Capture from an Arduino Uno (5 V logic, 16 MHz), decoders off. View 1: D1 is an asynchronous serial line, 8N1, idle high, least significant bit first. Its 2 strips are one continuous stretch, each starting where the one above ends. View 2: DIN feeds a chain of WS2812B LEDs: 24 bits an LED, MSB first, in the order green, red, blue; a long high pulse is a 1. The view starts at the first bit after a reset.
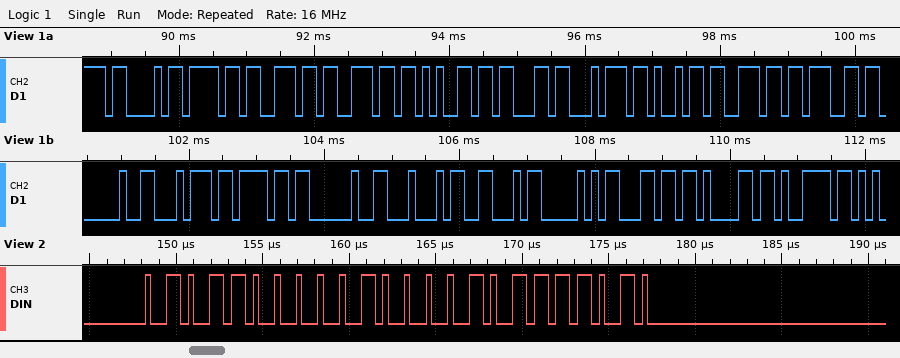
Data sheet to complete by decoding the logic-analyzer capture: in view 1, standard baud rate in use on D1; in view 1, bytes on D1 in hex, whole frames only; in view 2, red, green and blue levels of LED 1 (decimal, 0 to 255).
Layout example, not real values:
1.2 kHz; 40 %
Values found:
9600 baud; 43 6F 6E 6E 65 63 74 69 6E 67 20 74 6F 20 44 46 50 6C 61 79; 33, 88, 122
